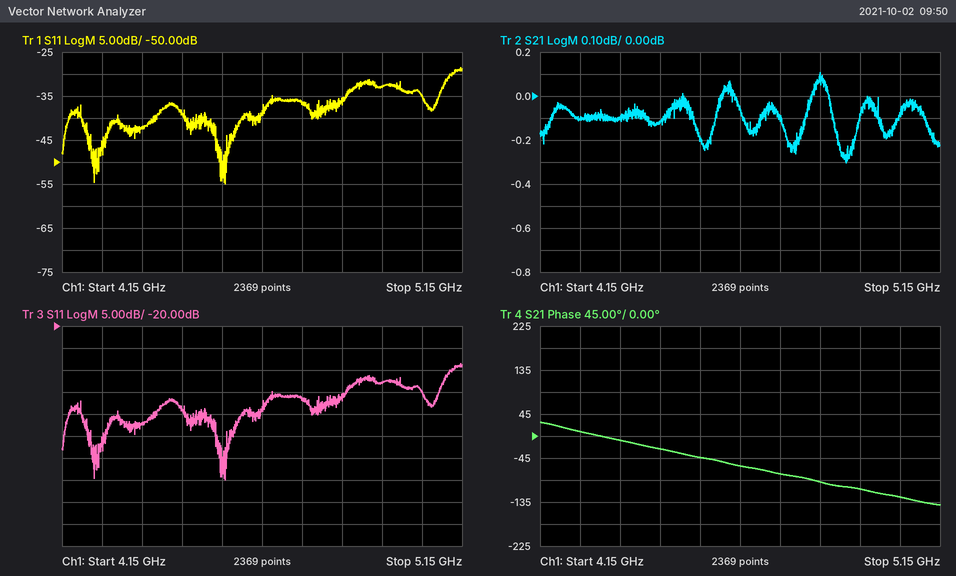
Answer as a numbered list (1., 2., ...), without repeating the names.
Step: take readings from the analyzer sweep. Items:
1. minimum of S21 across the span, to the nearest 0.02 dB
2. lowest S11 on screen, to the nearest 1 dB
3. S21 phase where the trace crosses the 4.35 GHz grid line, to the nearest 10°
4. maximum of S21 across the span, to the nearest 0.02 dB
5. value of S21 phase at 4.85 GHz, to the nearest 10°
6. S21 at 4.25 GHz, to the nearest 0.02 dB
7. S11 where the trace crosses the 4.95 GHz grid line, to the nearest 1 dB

1. -0.30 dB
2. -55 dB
3. -10°
4. 0.10 dB
5. -90°
6. -0.10 dB
7. -33 dB
